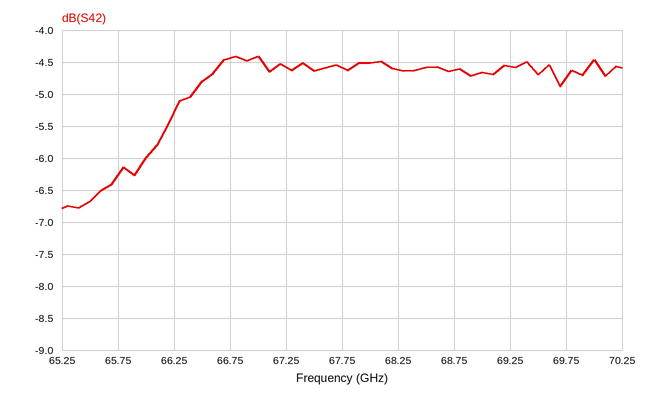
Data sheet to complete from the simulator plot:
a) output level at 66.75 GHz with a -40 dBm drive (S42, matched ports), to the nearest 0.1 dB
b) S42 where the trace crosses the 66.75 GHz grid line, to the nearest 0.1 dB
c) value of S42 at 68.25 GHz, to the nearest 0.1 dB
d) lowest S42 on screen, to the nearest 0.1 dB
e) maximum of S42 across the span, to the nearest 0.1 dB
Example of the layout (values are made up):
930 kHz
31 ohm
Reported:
-44.4 dBm
-4.4 dB
-4.6 dB
-6.8 dB
-4.4 dB
